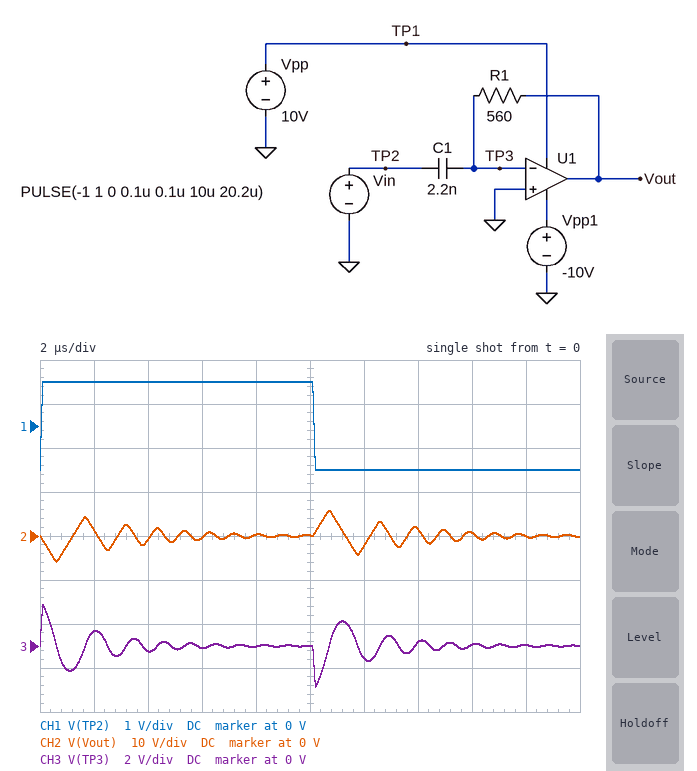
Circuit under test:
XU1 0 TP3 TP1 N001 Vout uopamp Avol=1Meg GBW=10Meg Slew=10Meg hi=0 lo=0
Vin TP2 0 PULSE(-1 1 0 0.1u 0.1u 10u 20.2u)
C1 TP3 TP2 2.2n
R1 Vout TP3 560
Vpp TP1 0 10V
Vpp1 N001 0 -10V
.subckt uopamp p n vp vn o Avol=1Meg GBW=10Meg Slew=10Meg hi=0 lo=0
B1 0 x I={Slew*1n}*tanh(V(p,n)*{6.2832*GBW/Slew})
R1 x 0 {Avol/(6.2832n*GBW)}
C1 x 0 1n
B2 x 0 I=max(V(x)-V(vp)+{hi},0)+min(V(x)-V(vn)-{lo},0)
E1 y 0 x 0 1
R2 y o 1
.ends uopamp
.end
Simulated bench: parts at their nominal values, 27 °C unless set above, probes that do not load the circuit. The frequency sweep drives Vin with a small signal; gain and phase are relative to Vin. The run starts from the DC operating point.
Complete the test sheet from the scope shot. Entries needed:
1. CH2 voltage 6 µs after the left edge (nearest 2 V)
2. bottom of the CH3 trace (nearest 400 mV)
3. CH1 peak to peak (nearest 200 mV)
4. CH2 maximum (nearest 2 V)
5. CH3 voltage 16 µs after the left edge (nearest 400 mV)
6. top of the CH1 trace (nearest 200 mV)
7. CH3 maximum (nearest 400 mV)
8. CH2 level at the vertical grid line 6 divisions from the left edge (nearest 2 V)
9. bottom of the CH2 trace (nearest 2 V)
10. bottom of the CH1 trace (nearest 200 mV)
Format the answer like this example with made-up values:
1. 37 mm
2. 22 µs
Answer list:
1. 0 V
2. -2.0 V
3. 2.0 V
4. 6 V
5. 0 V
6. 1.0 V
7. 2.0 V
8. -2 V
9. -6 V
10. -1.0 V
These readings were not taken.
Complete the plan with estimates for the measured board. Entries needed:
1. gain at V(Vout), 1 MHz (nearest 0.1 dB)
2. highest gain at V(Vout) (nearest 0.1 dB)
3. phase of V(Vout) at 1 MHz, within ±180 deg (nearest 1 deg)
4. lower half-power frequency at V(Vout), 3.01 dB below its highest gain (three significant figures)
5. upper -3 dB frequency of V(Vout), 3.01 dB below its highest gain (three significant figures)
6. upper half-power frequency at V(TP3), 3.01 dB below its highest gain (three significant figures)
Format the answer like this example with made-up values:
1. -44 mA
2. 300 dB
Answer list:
1. 30.0 dB
2. 37.8 dB
3. -114 deg
4. 1.07 MHz
5. 1.20 MHz
6. 1.21 MHz
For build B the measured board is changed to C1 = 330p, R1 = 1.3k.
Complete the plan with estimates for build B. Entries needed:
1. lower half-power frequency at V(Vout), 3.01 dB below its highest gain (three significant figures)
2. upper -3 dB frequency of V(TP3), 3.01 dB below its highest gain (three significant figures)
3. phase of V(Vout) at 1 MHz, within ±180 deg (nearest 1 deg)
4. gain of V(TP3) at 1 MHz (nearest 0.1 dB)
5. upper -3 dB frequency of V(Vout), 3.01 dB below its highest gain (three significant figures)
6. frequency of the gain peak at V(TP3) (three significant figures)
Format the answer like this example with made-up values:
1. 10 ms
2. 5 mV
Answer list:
1. 1.75 MHz
2. 2.17 MHz
3. -98 deg
4. -8.7 dB
5. 2.12 MHz
6. 1.94 MHz
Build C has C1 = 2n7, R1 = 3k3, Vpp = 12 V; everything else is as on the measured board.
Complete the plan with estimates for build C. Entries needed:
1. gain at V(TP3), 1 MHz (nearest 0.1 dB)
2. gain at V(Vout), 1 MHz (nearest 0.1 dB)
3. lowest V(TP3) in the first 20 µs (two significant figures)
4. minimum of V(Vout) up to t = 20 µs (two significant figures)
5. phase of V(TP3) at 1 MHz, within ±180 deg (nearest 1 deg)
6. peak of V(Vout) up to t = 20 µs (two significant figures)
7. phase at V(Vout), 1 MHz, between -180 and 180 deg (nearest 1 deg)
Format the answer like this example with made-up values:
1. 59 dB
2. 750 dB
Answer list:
1. 1.7 dB
2. 21.7 dB
3. -2.3 V
4. -10 V
5. 1 deg
6. 12 V
7. 91 deg
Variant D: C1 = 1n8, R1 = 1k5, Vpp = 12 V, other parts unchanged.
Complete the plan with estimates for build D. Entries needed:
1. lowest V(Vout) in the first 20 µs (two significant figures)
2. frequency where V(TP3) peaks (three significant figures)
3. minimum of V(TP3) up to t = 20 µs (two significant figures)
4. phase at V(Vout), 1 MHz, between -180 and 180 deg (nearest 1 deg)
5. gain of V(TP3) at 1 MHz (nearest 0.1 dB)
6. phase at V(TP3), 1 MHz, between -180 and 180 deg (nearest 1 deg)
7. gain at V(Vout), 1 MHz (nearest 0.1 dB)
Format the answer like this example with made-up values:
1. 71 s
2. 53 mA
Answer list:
1. -9.0 V
2. 769 kHz
3. -2.1 V
4. 98 deg
5. 7.6 dB
6. 8 deg
7. 27.6 dB
